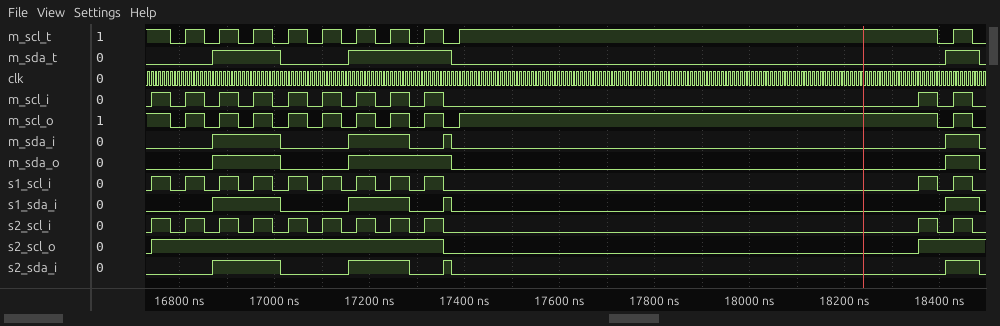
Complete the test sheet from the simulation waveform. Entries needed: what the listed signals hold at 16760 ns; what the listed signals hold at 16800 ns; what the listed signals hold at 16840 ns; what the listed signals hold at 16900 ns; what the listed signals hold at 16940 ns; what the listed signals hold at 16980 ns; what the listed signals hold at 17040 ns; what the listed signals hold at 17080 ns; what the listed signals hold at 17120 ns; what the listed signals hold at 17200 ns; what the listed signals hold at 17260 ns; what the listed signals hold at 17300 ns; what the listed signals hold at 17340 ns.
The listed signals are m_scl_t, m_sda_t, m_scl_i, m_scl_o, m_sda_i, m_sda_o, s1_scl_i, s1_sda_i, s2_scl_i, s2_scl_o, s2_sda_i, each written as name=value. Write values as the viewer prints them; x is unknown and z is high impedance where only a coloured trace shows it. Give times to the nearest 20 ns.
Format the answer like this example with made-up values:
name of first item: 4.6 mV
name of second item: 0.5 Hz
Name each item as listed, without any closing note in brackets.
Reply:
what the listed signals hold at 16760 ns: m_scl_t=1, m_sda_t=0, m_scl_i=1, m_scl_o=1, m_sda_i=0, m_sda_o=0, s1_scl_i=1, s1_sda_i=0, s2_scl_i=1, s2_scl_o=1, s2_sda_i=0
what the listed signals hold at 16800 ns: m_scl_t=0, m_sda_t=0, m_scl_i=0, m_scl_o=0, m_sda_i=0, m_sda_o=0, s1_scl_i=0, s1_sda_i=0, s2_scl_i=0, s2_scl_o=1, s2_sda_i=0
what the listed signals hold at 16840 ns: m_scl_t=1, m_sda_t=0, m_scl_i=1, m_scl_o=1, m_sda_i=0, m_sda_o=0, s1_scl_i=1, s1_sda_i=0, s2_scl_i=1, s2_scl_o=1, s2_sda_i=0
what the listed signals hold at 16900 ns: m_scl_t=1, m_sda_t=1, m_scl_i=1, m_scl_o=1, m_sda_i=1, m_sda_o=1, s1_scl_i=1, s1_sda_i=1, s2_scl_i=1, s2_scl_o=1, s2_sda_i=1
what the listed signals hold at 16940 ns: m_scl_t=0, m_sda_t=1, m_scl_i=0, m_scl_o=0, m_sda_i=1, m_sda_o=1, s1_scl_i=0, s1_sda_i=1, s2_scl_i=0, s2_scl_o=1, s2_sda_i=1
what the listed signals hold at 16980 ns: m_scl_t=1, m_sda_t=1, m_scl_i=1, m_scl_o=1, m_sda_i=1, m_sda_o=1, s1_scl_i=1, s1_sda_i=1, s2_scl_i=1, s2_scl_o=1, s2_sda_i=1
what the listed signals hold at 17040 ns: m_scl_t=1, m_sda_t=0, m_scl_i=1, m_scl_o=1, m_sda_i=0, m_sda_o=0, s1_scl_i=1, s1_sda_i=0, s2_scl_i=1, s2_scl_o=1, s2_sda_i=0
what the listed signals hold at 17080 ns: m_scl_t=0, m_sda_t=0, m_scl_i=0, m_scl_o=0, m_sda_i=0, m_sda_o=0, s1_scl_i=0, s1_sda_i=0, s2_scl_i=0, s2_scl_o=1, s2_sda_i=0
what the listed signals hold at 17120 ns: m_scl_t=1, m_sda_t=0, m_scl_i=1, m_scl_o=1, m_sda_i=0, m_sda_o=0, s1_scl_i=1, s1_sda_i=0, s2_scl_i=1, s2_scl_o=1, s2_sda_i=0
what the listed signals hold at 17200 ns: m_scl_t=1, m_sda_t=1, m_scl_i=1, m_scl_o=1, m_sda_i=1, m_sda_o=1, s1_scl_i=1, s1_sda_i=1, s2_scl_i=1, s2_scl_o=1, s2_sda_i=1
what the listed signals hold at 17260 ns: m_scl_t=1, m_sda_t=1, m_scl_i=1, m_scl_o=1, m_sda_i=1, m_sda_o=1, s1_scl_i=1, s1_sda_i=1, s2_scl_i=1, s2_scl_o=1, s2_sda_i=1
what the listed signals hold at 17300 ns: m_scl_t=0, m_sda_t=1, m_scl_i=0, m_scl_o=0, m_sda_i=0, m_sda_o=1, s1_scl_i=0, s1_sda_i=0, s2_scl_i=0, s2_scl_o=1, s2_sda_i=0
what the listed signals hold at 17340 ns: m_scl_t=1, m_sda_t=1, m_scl_i=1, m_scl_o=1, m_sda_i=0, m_sda_o=1, s1_scl_i=1, s1_sda_i=0, s2_scl_i=1, s2_scl_o=1, s2_sda_i=0
